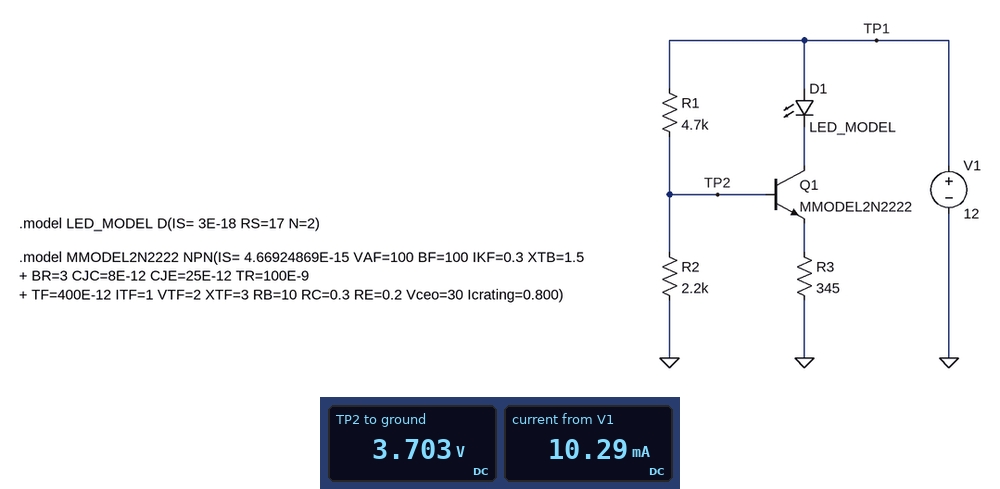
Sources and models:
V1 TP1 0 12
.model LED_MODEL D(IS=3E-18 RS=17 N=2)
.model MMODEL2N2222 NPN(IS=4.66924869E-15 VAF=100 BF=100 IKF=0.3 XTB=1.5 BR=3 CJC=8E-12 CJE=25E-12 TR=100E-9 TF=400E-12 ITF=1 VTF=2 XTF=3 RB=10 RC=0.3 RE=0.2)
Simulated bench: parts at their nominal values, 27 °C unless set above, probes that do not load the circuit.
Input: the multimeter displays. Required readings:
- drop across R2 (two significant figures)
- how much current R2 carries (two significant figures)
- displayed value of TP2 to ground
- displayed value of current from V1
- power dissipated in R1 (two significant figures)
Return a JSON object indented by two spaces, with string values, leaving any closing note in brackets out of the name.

{
  "drop across R2": "3.7 V",
  "how much current R2 carries": "1.7 mA",
  "displayed value of TP2 to ground": "3.703 V",
  "displayed value of current from V1": "10.29 mA",
  "power dissipated in R1": "15 mW"
}
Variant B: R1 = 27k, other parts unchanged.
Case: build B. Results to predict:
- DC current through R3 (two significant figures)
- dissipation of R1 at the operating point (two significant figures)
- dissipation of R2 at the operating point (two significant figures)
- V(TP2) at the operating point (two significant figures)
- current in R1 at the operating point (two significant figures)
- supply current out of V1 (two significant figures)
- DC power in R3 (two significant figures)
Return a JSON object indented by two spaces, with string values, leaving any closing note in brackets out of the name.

{
  "DC current through R3": "670 µA",
  "dissipation of R1 at the operating point": "4.6 mW",
  "dissipation of R2 at the operating point": "360 µW",
  "V(TP2) at the operating point": "890 mV",
  "current in R1 at the operating point": "410 µA",
  "supply current out of V1": "1.1 mA",
  "DC power in R3": "150 µW"
}
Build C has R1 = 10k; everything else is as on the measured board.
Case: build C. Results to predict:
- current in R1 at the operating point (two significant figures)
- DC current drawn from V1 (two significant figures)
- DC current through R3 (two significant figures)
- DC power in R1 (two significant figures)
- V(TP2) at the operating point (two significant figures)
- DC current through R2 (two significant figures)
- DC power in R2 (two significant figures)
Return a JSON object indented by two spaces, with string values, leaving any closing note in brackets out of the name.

{
  "current in R1 at the operating point": "990 µA",
  "DC current drawn from V1": "5.0 mA",
  "DC current through R3": "4.0 mA",
  "DC power in R1": "9.8 mW",
  "V(TP2) at the operating point": "2.1 V",
  "DC current through R2": "950 µA",
  "DC power in R2": "2.0 mW"
}
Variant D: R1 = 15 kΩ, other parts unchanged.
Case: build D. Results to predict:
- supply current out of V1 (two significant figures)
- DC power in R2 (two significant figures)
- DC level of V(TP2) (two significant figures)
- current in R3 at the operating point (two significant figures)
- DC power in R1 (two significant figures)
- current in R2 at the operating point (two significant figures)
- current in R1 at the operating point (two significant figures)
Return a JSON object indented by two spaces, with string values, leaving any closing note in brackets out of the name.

{
  "supply current out of V1": "3.0 mA",
  "DC power in R2": "1.0 mW",
  "DC level of V(TP2)": "1.5 V",
  "current in R3 at the operating point": "2.3 mA",
  "DC power in R1": "7.4 mW",
  "current in R2 at the operating point": "680 µA",
  "current in R1 at the operating point": "700 µA"
}
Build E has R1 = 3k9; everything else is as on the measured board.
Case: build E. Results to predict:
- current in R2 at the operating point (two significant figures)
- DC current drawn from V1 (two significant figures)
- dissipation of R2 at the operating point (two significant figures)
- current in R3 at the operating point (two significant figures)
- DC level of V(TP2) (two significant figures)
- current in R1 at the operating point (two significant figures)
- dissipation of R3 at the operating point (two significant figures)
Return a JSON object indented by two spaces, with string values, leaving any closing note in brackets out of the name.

{
  "current in R2 at the operating point": "1.9 mA",
  "DC current drawn from V1": "12 mA",
  "dissipation of R2 at the operating point": "8.0 mW",
  "current in R3 at the operating point": "10 mA",
  "DC level of V(TP2)": "4.2 V",
  "current in R1 at the operating point": "2.0 mA",
  "dissipation of R3 at the operating point": "35 mW"
}
